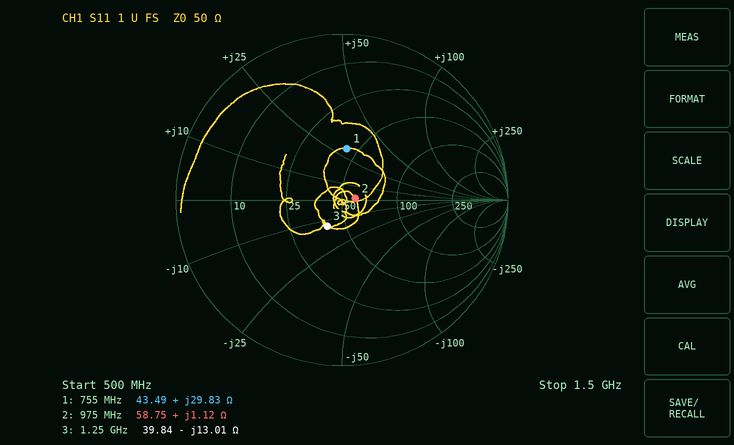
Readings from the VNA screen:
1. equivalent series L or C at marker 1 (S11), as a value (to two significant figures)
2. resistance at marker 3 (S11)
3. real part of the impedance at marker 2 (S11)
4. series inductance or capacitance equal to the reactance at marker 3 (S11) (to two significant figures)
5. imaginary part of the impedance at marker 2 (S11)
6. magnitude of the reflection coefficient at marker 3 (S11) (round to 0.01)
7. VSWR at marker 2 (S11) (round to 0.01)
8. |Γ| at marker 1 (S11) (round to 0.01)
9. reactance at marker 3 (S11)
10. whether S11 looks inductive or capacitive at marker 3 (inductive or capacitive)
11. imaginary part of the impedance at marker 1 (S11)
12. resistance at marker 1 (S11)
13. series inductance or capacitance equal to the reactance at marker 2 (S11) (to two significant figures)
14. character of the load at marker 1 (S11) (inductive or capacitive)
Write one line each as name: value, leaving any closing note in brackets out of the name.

equivalent series L or C at marker 1 (S11), as a value: 6.3 nH
resistance at marker 3: 39.84 Ω
real part of the impedance at marker 2: 58.75 Ω
series inductance or capacitance equal to the reactance at marker 3 (S11): 9.8 pF
imaginary part of the impedance at marker 2: +1.12 Ω
magnitude of the reflection coefficient at marker 3 (S11): 0.18
VSWR at marker 2 (S11): 1.18
|Γ| at marker 1 (S11): 0.31
reactance at marker 3: -13.01 Ω
whether S11 looks inductive or capacitive at marker 3: capacitive
imaginary part of the impedance at marker 1: +29.83 Ω
resistance at marker 1: 43.49 Ω
series inductance or capacitance equal to the reactance at marker 2 (S11): 180 pH
character of the load at marker 1 (S11): inductive
